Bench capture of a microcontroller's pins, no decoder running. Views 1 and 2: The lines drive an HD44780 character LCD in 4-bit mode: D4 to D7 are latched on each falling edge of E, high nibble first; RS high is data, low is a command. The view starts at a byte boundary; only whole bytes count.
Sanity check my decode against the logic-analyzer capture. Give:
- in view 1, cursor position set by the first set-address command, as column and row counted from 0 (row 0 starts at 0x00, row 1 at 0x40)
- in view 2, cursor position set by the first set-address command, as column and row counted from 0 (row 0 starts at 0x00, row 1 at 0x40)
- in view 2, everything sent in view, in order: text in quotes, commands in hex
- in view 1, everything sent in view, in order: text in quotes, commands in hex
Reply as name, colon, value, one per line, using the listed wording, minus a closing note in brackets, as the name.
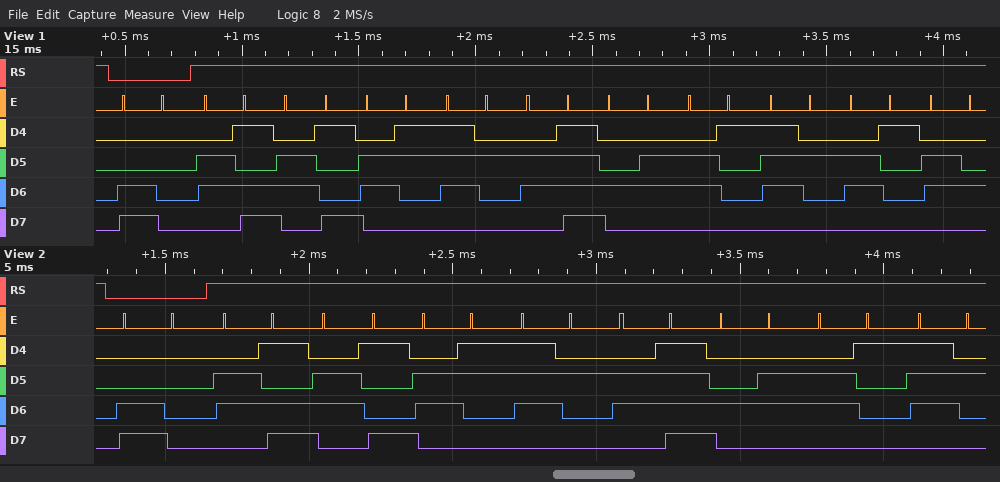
in view 1, cursor position set by the first set-address command, as column and row counted from 0: column 0, row 1
in view 2, cursor position set by the first set-address command, as column and row counted from 0: column 0, row 1
in view 2, everything sent in view, in order: text in quotes, commands in hex: 0xC0 "microFar"
in view 1, everything sent in view, in order: text in quotes, commands in hex: 0xC0 "microFarad"
